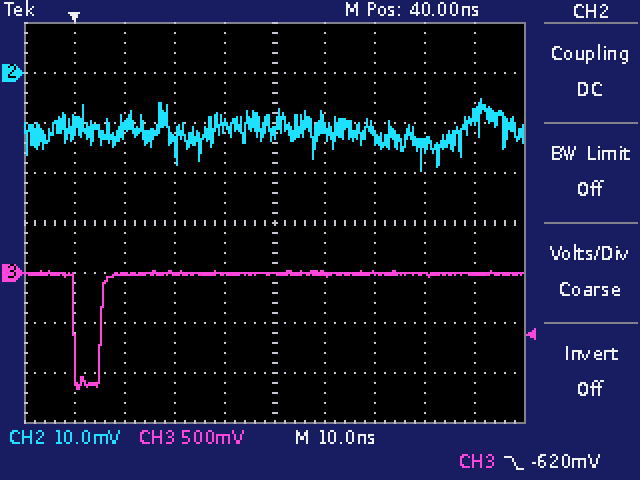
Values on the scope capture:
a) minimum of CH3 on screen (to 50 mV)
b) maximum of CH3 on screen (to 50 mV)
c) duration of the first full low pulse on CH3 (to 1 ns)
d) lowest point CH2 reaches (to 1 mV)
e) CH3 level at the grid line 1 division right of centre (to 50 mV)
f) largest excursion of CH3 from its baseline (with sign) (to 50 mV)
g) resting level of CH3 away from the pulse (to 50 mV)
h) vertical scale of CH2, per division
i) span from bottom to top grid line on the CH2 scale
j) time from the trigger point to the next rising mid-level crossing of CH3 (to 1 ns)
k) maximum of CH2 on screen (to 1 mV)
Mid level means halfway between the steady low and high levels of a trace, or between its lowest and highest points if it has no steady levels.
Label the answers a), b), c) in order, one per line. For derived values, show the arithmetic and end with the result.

a) -1.15 V
b) 0 mV
c) 5 ns
d) -20 mV
e) 0 mV
f) -1.15 V − (0 mV) = -1.15 V
g) 0 mV
h) 10 mV
i) 80 mV
j) 5 ns
k) -5 mV
